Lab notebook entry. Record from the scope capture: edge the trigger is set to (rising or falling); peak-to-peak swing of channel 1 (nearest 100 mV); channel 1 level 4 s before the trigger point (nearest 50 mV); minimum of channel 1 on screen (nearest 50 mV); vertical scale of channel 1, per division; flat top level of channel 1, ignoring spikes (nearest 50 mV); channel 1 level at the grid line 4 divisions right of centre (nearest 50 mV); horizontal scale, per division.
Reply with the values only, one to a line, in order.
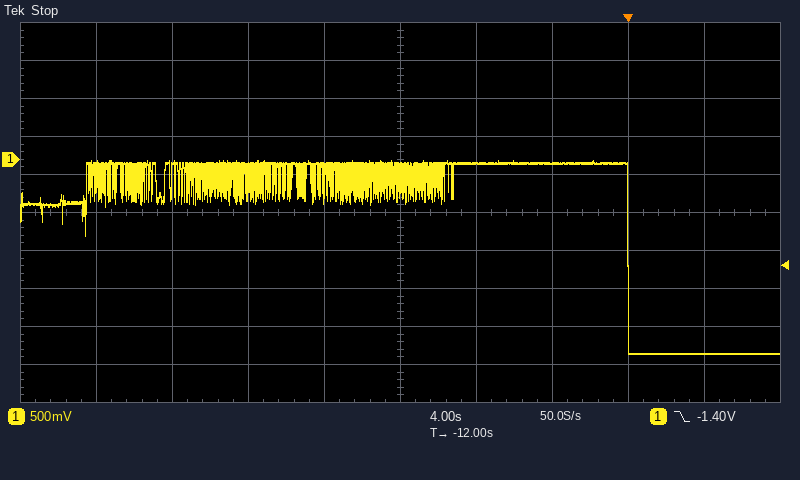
falling
2.50 V
-50 mV
-2.55 V
500 mV
-50 mV
-2.55 V
4 s
